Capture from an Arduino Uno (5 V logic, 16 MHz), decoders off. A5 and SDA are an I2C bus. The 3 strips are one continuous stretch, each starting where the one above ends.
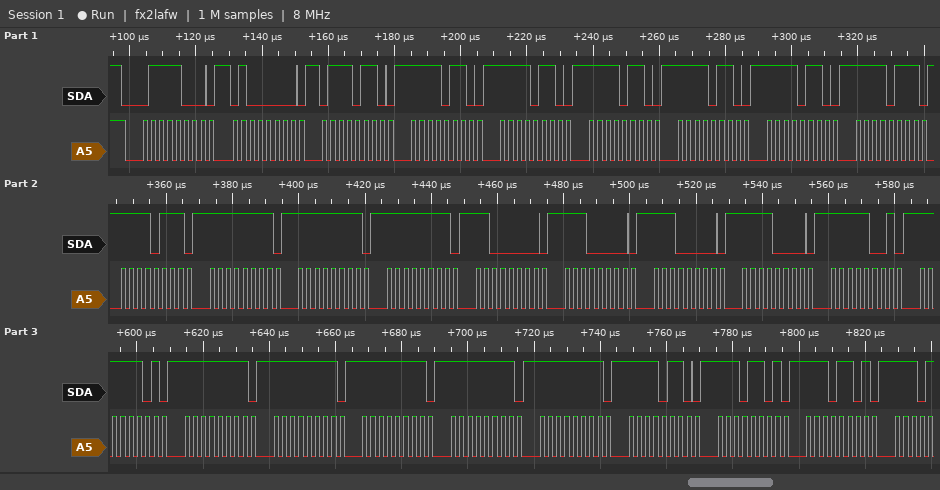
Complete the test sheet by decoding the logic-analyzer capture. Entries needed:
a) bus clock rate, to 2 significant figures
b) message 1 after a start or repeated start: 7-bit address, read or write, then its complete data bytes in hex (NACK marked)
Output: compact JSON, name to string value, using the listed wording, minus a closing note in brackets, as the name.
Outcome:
{"bus clock rate, to 2 significant figures": "400 kHz", "message 1 after a start or repeated start: 7-bit address, read or write, then its complete data bytes in hex": "0x3C write: 40 76 F6 F6 F6 F6 F6 F7 F7 FF FF FF C0 E0 E0 F0 F9 FD FF FF FF FF FF F6 ED ED"}
